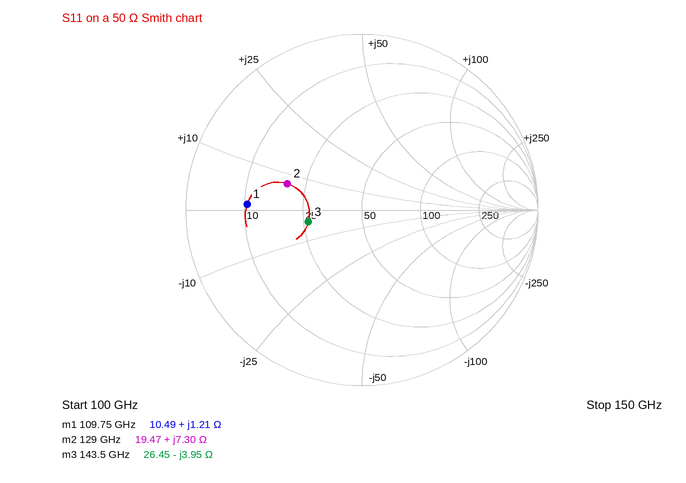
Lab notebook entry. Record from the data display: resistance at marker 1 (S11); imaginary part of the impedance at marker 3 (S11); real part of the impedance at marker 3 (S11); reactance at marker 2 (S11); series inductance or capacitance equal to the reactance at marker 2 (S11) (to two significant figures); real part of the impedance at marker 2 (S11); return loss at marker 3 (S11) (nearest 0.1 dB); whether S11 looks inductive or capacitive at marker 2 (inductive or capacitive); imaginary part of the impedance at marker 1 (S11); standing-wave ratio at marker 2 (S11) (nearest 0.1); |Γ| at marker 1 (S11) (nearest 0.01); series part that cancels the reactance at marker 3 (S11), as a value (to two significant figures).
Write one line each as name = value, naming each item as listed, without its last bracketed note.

resistance at marker 1 = 10.49 Ω
imaginary part of the impedance at marker 3 = -3.95 Ω
real part of the impedance at marker 3 = 26.45 Ω
reactance at marker 2 = +7.30 Ω
series inductance or capacitance equal to the reactance at marker 2 (S11) = 9.0 pH
real part of the impedance at marker 2 = 19.47 Ω
return loss at marker 3 (S11) = 10.1 dB
whether S11 looks inductive or capacitive at marker 2 = inductive
imaginary part of the impedance at marker 1 = +1.21 Ω
standing-wave ratio at marker 2 (S11) = 2.6
|Γ| at marker 1 (S11) = 0.65
series part that cancels the reactance at marker 3 (S11), as a value = 4.4 pH
